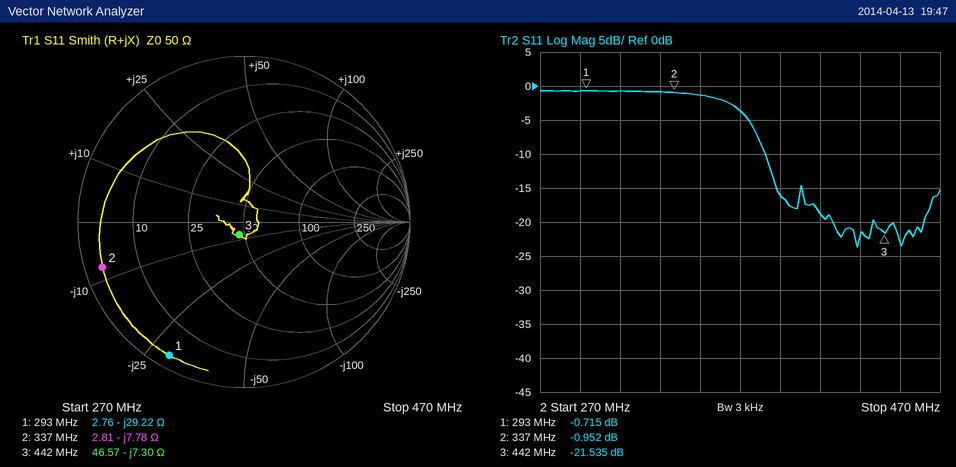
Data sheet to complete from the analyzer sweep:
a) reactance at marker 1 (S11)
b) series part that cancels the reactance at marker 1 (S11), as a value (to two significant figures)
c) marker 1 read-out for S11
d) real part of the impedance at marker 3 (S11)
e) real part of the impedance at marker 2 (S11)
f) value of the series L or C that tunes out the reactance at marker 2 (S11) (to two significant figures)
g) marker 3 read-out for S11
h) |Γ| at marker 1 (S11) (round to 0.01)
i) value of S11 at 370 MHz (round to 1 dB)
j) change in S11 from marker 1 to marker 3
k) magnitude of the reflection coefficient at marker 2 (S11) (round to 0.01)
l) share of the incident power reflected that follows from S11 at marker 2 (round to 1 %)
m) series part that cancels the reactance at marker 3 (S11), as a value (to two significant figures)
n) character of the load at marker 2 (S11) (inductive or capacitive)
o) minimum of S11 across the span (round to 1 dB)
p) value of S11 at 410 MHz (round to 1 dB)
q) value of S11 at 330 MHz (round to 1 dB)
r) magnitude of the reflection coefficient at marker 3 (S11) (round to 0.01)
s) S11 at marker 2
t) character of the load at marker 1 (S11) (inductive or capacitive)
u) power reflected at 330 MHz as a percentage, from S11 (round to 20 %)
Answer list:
-29.22 Ω
16 nH
-0.715 dB
46.57 Ω
2.81 Ω
3.7 nH
-21.535 dB
0.92
-4 dB
-20.820 dB
0.90
80 %
2.6 nH
capacitive
-24 dB
-19 dB
-1 dB
0.08
-0.952 dB
capacitive
80 %
